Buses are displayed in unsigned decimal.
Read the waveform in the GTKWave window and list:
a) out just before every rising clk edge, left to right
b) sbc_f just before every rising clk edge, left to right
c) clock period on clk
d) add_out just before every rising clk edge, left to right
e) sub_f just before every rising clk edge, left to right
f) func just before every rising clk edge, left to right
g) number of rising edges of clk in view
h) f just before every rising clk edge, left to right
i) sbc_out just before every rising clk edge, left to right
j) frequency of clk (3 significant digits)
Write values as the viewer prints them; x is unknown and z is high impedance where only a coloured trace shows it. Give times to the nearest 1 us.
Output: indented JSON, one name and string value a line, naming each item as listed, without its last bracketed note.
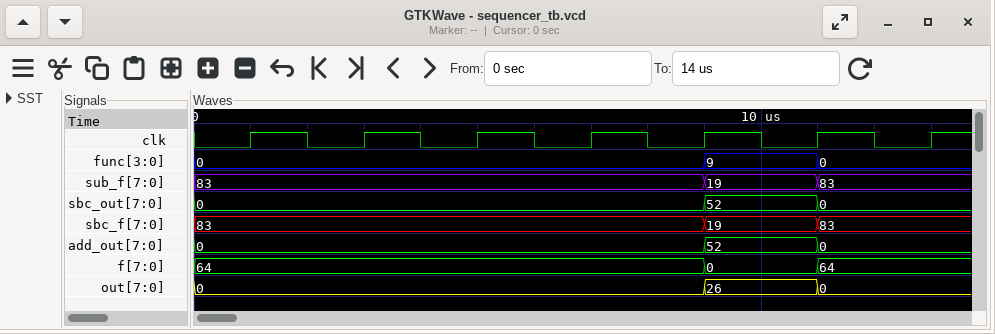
{
  "out just before every rising clk edge, left to right": "0, 0, 0, 0, 0, 26, 0",
  "sbc_f just before every rising clk edge, left to right": "83, 83, 83, 83, 83, 19, 83",
  "clock period on clk": "2 us",
  "add_out just before every rising clk edge, left to right": "0, 0, 0, 0, 0, 52, 0",
  "sub_f just before every rising clk edge, left to right": "83, 83, 83, 83, 83, 19, 83",
  "func just before every rising clk edge, left to right": "0, 0, 0, 0, 0, 9, 0",
  "number of rising edges of clk in view": "7",
  "f just before every rising clk edge, left to right": "64, 64, 64, 64, 64, 0, 64",
  "sbc_out just before every rising clk edge, left to right": "0, 0, 0, 0, 0, 52, 0",
  "frequency of clk": "500 kHz"
}
